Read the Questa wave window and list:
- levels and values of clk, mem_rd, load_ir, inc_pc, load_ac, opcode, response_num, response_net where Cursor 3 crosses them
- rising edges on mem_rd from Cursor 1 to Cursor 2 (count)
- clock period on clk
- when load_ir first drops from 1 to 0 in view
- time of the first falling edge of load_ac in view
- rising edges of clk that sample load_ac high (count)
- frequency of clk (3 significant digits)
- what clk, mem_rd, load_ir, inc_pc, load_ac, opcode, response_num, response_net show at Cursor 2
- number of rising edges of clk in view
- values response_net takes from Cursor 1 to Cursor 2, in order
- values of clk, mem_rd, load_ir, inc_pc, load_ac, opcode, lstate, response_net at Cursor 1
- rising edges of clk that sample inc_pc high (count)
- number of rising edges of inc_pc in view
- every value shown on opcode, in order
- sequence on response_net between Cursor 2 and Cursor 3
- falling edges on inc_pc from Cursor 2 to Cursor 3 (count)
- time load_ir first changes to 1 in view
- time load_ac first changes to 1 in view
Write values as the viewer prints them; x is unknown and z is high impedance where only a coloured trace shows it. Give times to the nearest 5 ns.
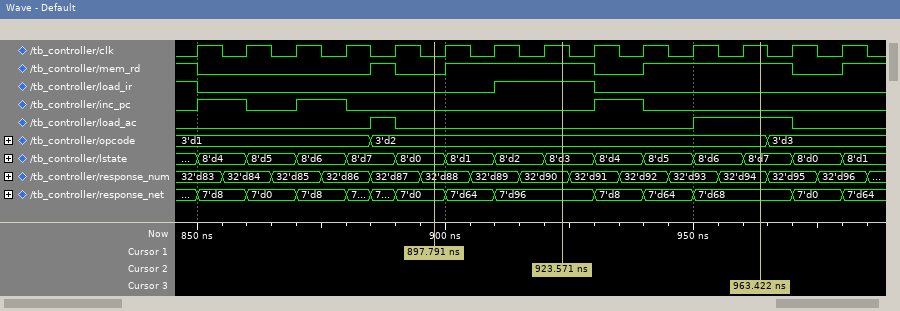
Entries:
clk=1, mem_rd=1, load_ir=0, inc_pc=0, load_ac=1, opcode=3'd2, response_num=32'd94, response_net=7'd68
1
10 ns
850 ns
890 ns
3
100 MHz
clk=1, mem_rd=1, load_ir=1, inc_pc=0, load_ac=0, opcode=3'd2, response_num=32'd90, response_net=7'd96
14
7'd0, 7'd64, 7'd96
clk=0, mem_rd=0, load_ir=0, inc_pc=0, load_ac=0, opcode=3'd2, lstate=8'd0, response_net=7'd0
3
3
3'd1, 3'd2, 3'd3
7'd96, 7'd8, 7'd64, 7'd68
1
910 ns
885 ns
